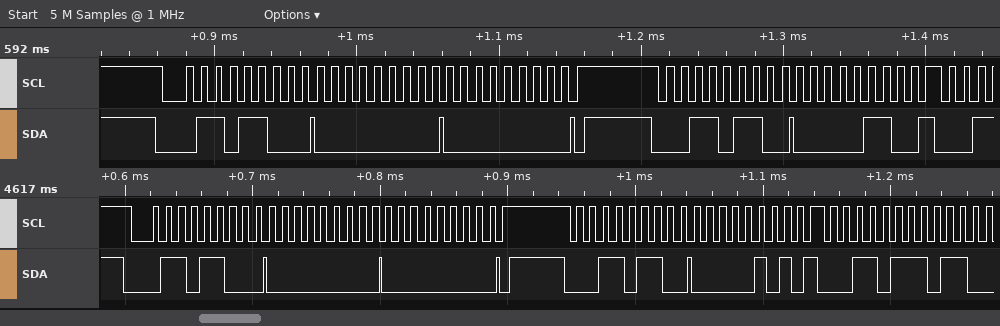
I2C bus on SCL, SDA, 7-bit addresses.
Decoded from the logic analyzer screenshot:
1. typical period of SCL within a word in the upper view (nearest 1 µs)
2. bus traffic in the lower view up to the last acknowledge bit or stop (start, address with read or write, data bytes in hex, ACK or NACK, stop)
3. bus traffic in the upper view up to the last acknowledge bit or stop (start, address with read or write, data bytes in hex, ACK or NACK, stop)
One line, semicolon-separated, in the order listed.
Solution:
10 µs; start, address 36 write ACK, 00 ACK, 00 ACK, stop, start, address 1B write ACK, 05 ACK, repeated start, address 1B read ACK; start, address 36 write ACK, 00 ACK, 00 ACK, stop, start, address 1B write ACK, 06 ACK
